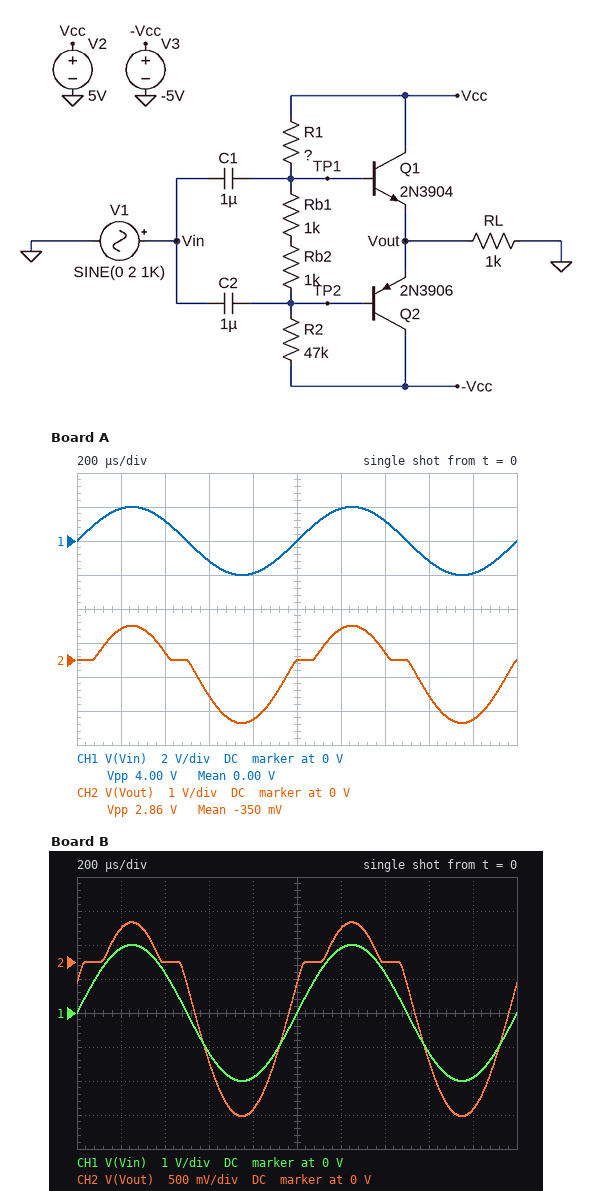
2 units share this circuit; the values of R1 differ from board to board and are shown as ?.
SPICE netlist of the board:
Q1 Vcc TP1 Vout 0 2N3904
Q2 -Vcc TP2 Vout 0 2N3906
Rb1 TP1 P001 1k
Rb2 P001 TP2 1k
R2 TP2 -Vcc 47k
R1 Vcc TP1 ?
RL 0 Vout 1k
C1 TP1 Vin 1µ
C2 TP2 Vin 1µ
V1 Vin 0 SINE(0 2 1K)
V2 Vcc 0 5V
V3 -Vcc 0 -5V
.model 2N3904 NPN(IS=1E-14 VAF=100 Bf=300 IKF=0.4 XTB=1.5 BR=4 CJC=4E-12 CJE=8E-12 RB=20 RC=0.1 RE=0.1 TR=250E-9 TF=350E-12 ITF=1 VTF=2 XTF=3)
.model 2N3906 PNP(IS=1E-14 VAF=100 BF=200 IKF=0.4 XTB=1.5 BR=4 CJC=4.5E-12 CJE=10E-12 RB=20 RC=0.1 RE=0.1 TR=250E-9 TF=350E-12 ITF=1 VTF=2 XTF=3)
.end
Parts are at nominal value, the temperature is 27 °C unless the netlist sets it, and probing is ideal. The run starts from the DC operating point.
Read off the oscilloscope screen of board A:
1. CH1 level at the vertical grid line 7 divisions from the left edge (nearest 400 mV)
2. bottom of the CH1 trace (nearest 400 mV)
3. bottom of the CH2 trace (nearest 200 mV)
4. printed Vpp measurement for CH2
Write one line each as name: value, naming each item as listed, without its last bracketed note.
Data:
CH1 level at the vertical grid line 7 divisions from the left edge: 1.2 V
bottom of the CH1 trace: -2.0 V
bottom of the CH2 trace: -1.8 V
printed Vpp measurement for CH2: 2.86 V
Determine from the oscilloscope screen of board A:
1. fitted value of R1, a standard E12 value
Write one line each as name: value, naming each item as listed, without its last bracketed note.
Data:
fitted value of R1, a standard E12 value: 56 kΩ
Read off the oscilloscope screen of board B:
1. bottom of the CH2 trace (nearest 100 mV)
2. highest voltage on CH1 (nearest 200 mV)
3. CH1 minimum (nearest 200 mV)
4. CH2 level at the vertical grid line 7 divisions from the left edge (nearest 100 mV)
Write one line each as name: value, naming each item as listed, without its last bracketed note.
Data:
bottom of the CH2 trace: -2.3 V
highest voltage on CH1: 2.0 V
CH1 minimum: -2.0 V
CH2 level at the vertical grid line 7 divisions from the left edge: 0 V
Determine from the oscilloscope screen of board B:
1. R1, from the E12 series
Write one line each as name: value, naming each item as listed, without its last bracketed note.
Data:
R1, from the E12 series: 68 kΩ
